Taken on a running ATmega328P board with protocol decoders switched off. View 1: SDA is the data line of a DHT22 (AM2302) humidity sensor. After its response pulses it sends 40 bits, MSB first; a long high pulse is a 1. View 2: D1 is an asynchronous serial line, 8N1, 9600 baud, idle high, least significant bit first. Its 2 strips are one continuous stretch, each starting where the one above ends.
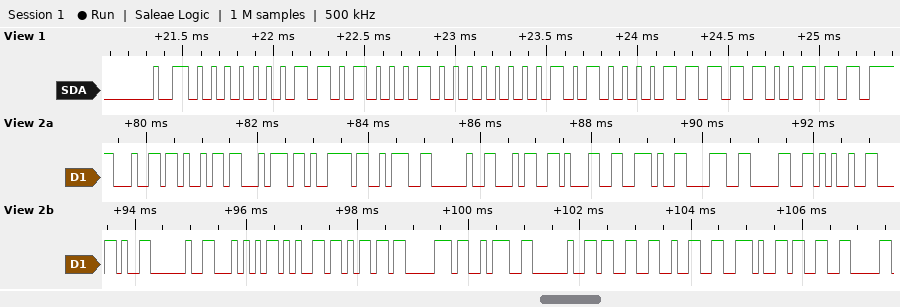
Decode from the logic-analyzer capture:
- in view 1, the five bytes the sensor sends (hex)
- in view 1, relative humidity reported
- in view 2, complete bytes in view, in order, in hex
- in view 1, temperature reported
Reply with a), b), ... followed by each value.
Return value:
a) 01 A2 01 43 E7
b) 41.8 %
c) 64 69 74 79 3A 20 34 31 2E 38 30 25 2C 20 54 65 6D 70 3A 20 33 32 2E 33
d) 32.3 °C
